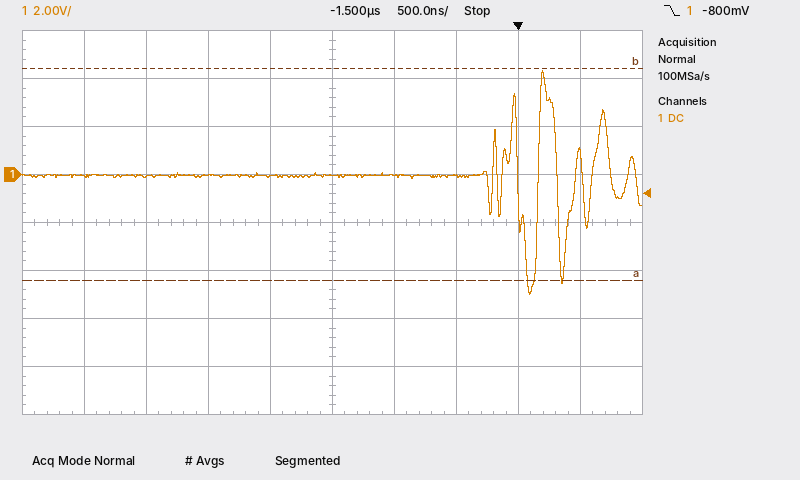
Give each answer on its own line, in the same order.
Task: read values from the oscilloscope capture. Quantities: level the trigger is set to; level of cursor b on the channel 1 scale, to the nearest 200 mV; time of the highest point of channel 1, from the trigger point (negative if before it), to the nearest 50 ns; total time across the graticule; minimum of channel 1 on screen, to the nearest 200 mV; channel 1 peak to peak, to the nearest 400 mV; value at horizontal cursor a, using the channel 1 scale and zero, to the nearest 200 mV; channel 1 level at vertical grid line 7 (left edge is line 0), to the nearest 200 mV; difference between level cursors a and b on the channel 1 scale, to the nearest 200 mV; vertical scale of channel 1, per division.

-800 mV
4.4 V
+200 ns
5 µs
-5.0 V
9.2 V
-4.4 V
0.0 V
8.8 V
2 V
